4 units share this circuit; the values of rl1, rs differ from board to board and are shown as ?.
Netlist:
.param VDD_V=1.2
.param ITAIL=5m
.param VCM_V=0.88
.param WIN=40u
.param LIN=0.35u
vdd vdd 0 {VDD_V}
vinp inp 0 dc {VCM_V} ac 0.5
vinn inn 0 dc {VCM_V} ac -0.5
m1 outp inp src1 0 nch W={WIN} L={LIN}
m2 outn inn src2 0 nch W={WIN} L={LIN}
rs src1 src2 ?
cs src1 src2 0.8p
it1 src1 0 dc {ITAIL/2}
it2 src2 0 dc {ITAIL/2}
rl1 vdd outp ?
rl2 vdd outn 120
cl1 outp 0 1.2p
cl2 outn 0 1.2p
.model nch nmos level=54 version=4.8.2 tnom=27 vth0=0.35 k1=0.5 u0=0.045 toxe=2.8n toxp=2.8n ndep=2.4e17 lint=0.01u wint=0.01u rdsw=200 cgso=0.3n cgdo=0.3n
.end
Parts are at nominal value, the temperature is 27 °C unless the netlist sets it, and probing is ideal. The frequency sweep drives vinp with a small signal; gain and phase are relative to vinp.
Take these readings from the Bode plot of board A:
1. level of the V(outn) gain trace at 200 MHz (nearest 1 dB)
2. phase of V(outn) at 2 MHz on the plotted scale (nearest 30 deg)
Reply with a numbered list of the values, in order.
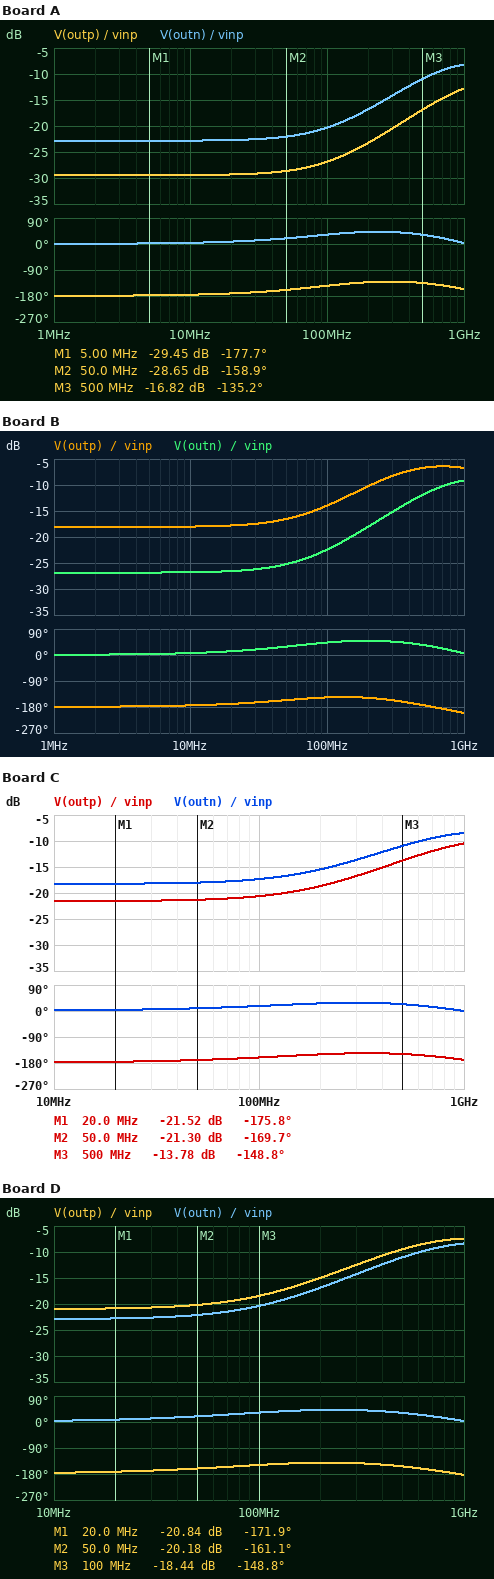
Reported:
1. -17 dB
2. 0 deg
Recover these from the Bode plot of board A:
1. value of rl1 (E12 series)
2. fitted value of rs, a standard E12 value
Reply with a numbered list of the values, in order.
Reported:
1. 56 Ω
2. 1.8 kΩ
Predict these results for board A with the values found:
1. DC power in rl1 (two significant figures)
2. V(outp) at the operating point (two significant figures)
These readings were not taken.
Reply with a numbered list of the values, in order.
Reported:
1. 350 µW
2. 1.1 V
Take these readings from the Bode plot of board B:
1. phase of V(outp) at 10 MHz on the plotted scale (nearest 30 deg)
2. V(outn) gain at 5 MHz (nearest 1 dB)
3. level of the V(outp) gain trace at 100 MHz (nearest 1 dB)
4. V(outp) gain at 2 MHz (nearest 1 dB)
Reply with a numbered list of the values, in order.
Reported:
1. -180 deg
2. -27 dB
3. -14 dB
4. -18 dB
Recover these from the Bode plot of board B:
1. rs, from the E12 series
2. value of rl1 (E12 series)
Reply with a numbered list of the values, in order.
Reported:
1. 2.7 kΩ
2. 330 Ω
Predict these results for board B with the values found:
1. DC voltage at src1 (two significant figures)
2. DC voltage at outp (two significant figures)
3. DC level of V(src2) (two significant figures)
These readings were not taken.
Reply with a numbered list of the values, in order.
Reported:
1. 26 mV
2. 380 mV
3. 52 mV
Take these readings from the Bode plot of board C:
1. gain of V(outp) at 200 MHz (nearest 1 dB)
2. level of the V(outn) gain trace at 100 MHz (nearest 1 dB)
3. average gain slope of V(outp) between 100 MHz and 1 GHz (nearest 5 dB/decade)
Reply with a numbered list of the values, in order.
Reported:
1. -19 dB
2. -17 dB
3. 10 dB/decade
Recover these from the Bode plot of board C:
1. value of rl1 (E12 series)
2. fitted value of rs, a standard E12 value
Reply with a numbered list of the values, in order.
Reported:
1. 82 Ω
2. 1 kΩ
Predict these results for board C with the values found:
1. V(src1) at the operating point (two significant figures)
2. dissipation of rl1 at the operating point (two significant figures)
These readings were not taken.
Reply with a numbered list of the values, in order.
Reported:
1. 55 mV
2. 510 µW
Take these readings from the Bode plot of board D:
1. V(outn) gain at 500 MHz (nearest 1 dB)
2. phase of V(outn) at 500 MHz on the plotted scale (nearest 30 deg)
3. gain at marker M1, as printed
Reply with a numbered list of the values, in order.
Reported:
1. -11 dB
2. 30 deg
3. -20.84 dB
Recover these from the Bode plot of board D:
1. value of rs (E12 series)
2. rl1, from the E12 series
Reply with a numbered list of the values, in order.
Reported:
1. 1.8 kΩ
2. 150 Ω
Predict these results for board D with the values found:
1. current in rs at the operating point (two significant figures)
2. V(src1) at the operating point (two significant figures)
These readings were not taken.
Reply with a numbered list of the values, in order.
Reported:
1. 1.2 µA
2. 50 mV
